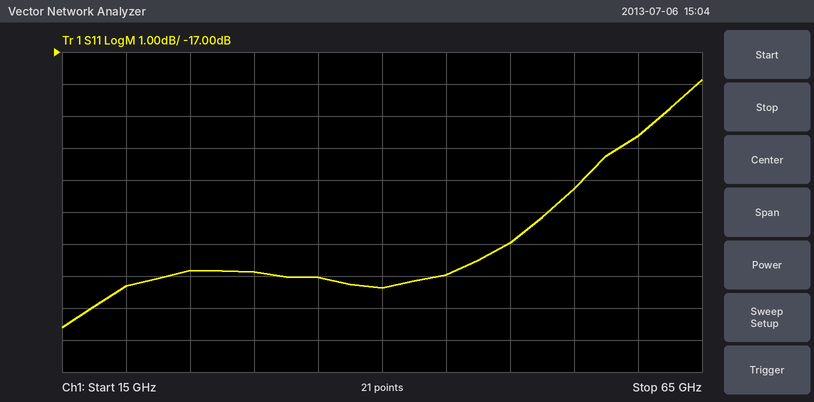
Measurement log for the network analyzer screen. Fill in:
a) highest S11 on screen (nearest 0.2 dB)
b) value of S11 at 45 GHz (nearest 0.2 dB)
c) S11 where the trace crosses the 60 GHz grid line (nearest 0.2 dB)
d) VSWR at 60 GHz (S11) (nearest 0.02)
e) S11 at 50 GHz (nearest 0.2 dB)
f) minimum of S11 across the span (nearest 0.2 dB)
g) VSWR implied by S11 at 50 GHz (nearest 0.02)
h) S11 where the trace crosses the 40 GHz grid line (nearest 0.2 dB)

-17.8 dB
-24.0 dB
-19.6 dB
1.24
-23.0 dB
-25.6 dB
1.16
-24.4 dB
